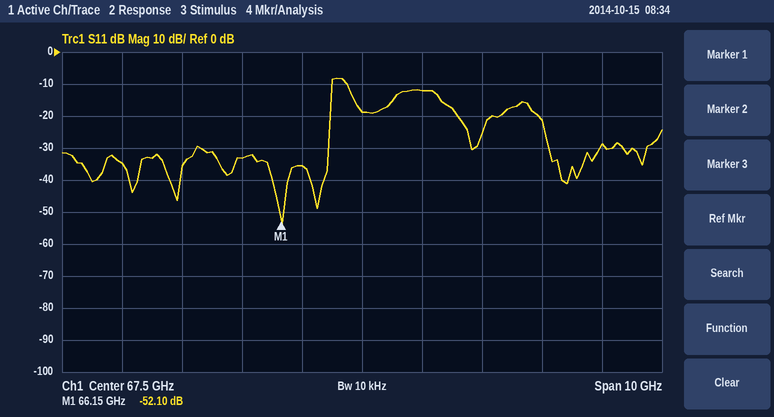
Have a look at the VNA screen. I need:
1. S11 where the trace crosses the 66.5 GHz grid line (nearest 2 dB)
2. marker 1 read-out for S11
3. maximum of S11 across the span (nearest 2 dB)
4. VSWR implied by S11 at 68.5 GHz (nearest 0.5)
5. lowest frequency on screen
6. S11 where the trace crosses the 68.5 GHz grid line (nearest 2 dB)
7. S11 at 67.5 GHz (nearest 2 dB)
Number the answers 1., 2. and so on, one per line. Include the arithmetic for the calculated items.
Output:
1. -36 dB
2. -52.10 dB
3. -8 dB
4. |Γ| = 10^(-12/20) = 0.2512; VSWR = (1 + 0.2512)/(1 − 0.2512) ≈ 1.67, so 1.5 to the nearest 0.5
5. 62.5 GHz
6. -12 dB
7. -18 dB
